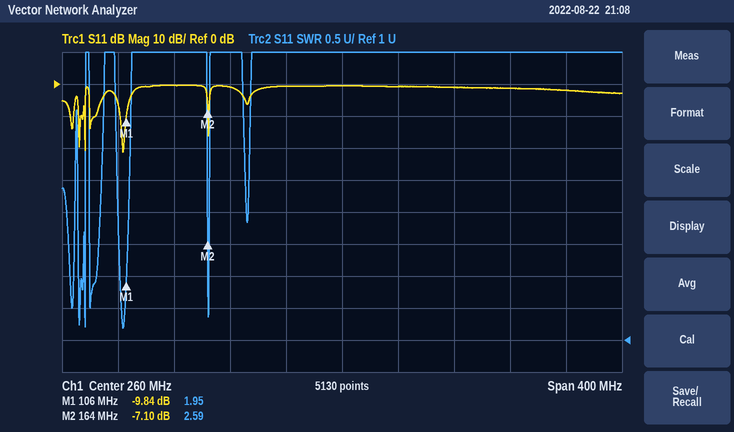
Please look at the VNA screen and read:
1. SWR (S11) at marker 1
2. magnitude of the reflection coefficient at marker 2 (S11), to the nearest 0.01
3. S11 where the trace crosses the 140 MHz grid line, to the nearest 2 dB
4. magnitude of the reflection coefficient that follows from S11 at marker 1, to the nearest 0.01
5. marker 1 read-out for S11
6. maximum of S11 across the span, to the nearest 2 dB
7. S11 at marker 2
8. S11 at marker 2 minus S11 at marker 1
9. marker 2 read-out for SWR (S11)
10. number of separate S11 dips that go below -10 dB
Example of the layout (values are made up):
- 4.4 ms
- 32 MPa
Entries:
- 1.95
- 0.44
- 0 dB
- 0.32
- -9.84 dB
- 0 dB
- -7.10 dB
- 2.74 dB
- 2.59
- 6
